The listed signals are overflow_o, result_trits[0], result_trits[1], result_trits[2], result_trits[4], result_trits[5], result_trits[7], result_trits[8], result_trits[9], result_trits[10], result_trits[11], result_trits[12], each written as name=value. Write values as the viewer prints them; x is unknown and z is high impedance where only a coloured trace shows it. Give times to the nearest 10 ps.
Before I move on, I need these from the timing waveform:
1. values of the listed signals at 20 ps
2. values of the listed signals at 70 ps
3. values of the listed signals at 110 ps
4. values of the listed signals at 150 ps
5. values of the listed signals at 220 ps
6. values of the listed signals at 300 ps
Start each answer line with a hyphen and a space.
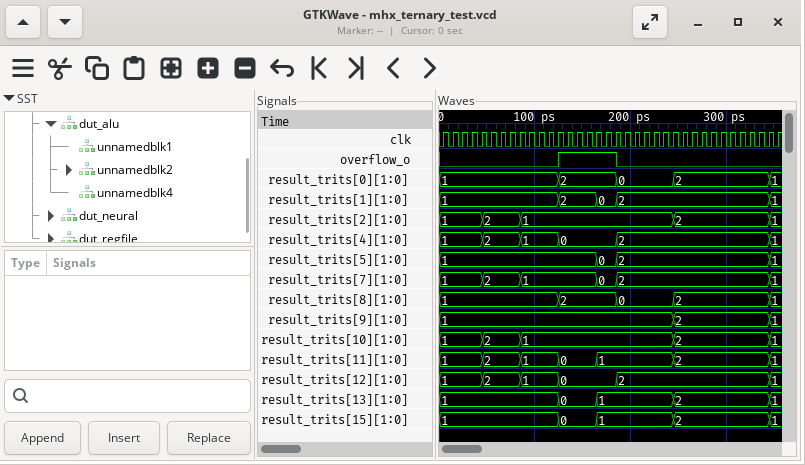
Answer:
- overflow_o=0, result_trits[0]=1, result_trits[1]=1, result_trits[2]=1, result_trits[4]=1, result_trits[5]=1, result_trits[7]=1, result_trits[8]=1, result_trits[9]=1, result_trits[10]=1, result_trits[11]=1, result_trits[12]=1
- overflow_o=0, result_trits[0]=1, result_trits[1]=1, result_trits[2]=2, result_trits[4]=2, result_trits[5]=1, result_trits[7]=2, result_trits[8]=1, result_trits[9]=1, result_trits[10]=2, result_trits[11]=2, result_trits[12]=2
- overflow_o=0, result_trits[0]=1, result_trits[1]=1, result_trits[2]=1, result_trits[4]=1, result_trits[5]=1, result_trits[7]=1, result_trits[8]=1, result_trits[9]=1, result_trits[10]=1, result_trits[11]=1, result_trits[12]=1
- overflow_o=1, result_trits[0]=2, result_trits[1]=2, result_trits[2]=1, result_trits[4]=0, result_trits[5]=1, result_trits[7]=1, result_trits[8]=2, result_trits[9]=1, result_trits[10]=1, result_trits[11]=0, result_trits[12]=0
- overflow_o=0, result_trits[0]=0, result_trits[1]=2, result_trits[2]=1, result_trits[4]=2, result_trits[5]=2, result_trits[7]=2, result_trits[8]=0, result_trits[9]=1, result_trits[10]=1, result_trits[11]=1, result_trits[12]=2
- overflow_o=0, result_trits[0]=2, result_trits[1]=2, result_trits[2]=2, result_trits[4]=2, result_trits[5]=2, result_trits[7]=2, result_trits[8]=2, result_trits[9]=2, result_trits[10]=2, result_trits[11]=2, result_trits[12]=2
